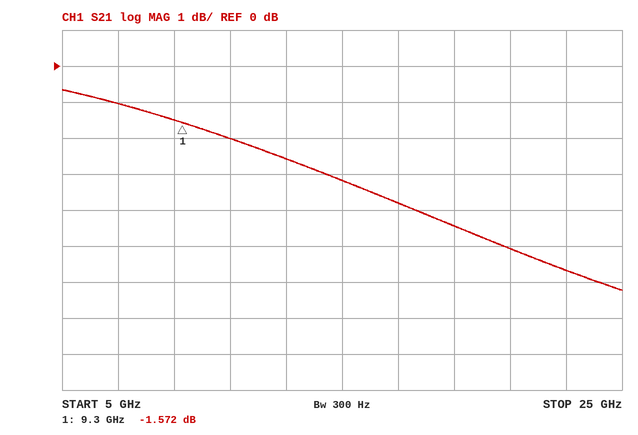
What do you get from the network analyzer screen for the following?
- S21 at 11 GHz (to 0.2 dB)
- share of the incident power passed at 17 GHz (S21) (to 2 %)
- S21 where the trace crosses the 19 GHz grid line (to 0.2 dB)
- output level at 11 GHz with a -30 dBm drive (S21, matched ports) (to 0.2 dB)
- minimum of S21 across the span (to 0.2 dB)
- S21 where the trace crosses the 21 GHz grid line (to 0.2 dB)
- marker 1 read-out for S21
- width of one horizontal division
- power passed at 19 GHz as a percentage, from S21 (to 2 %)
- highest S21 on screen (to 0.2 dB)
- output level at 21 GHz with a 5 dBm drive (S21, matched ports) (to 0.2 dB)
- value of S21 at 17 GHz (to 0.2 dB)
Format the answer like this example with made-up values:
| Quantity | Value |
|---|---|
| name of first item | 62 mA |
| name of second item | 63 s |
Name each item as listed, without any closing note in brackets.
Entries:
| Quantity | Value |
|---|---|
| S21 at 11 GHz | -2.0 dB |
| share of the incident power passed at 17 GHz (S21) | 42 % |
| S21 where the trace crosses the 19 GHz grid line | -4.4 dB |
| output level at 11 GHz with a -30 dBm drive (S21, matched ports) | -32.0 dBm |
| minimum of S21 across the span | -6.2 dB |
| S21 where the trace crosses the 21 GHz grid line | -5.0 dB |
| marker 1 read-out for S21 | -1.572 dB |
| width of one horizontal division | 2 GHz |
| power passed at 19 GHz as a percentage, from S21 | 36 % |
| highest S21 on screen | -0.6 dB |
| output level at 21 GHz with a 5 dBm drive (S21, matched ports) | 0.0 dBm |
| value of S21 at 17 GHz | -3.8 dB |
